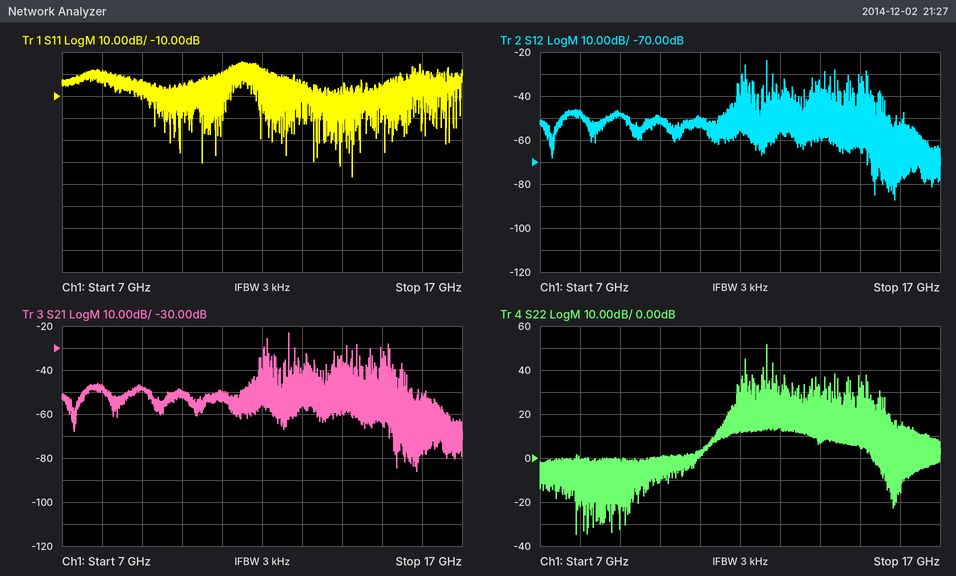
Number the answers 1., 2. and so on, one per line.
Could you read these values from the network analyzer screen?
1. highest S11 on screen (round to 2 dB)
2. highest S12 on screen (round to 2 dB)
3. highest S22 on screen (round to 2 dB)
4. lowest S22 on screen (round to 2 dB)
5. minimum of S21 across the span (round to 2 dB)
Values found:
1. 6 dB
2. -24 dB
3. 52 dB
4. -34 dB
5. -86 dB
